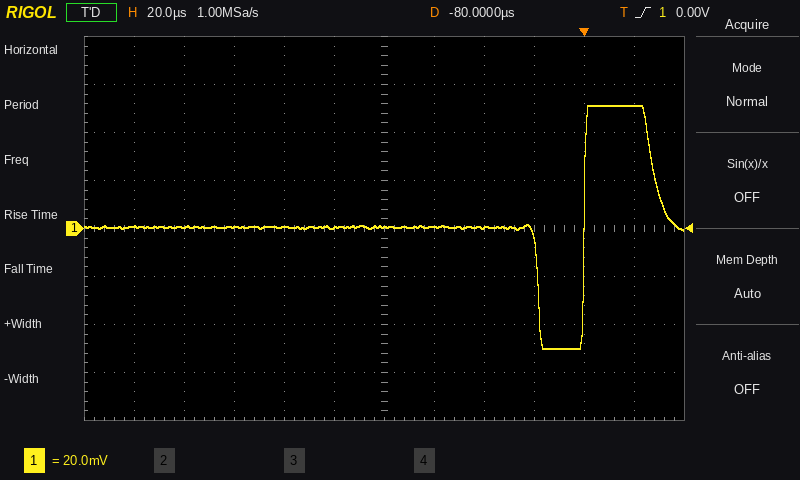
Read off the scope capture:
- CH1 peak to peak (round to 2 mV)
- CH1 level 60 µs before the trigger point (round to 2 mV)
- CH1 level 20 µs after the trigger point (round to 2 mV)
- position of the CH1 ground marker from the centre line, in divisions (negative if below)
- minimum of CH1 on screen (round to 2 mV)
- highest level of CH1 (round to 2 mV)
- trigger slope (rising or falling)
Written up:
102 mV
0 mV
52 mV
0.0 div
-50 mV
52 mV
rising
